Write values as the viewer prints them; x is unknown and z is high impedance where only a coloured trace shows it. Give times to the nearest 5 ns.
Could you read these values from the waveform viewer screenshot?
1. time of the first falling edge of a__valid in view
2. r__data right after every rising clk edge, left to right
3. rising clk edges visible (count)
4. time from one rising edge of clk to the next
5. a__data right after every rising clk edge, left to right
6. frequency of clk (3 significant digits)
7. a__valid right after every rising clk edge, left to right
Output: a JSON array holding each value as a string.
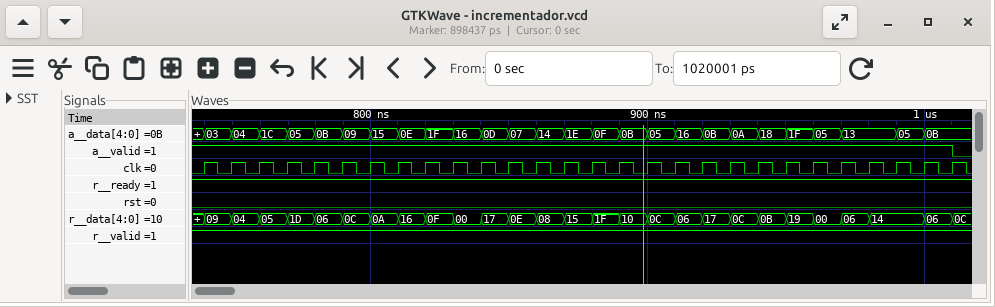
["1010 ns", "09, 04, 05, 1D, 06, 0C, 0A, 16, 0F, 00, 17, 0E, 08, 15, 1F, 10, 0C, 06, 17, 0C, 0B, 19, 00, 06, 14, 14, 06, 0C", "28", "10 ns", "03, 04, 1C, 05, 0B, 09, 15, 0E, 1F, 16, 0D, 07, 14, 1E, 0F, 0B, 05, 16, 0B, 0A, 18, 1F, 05, 13, 13, 05, 0B, 0B", "100 MHz", "1 1 1 1 1 1 1 1 1 1 1 1 1 1 1 1 1 1 1 1 1 1 1 1 1 1 1 0"]
